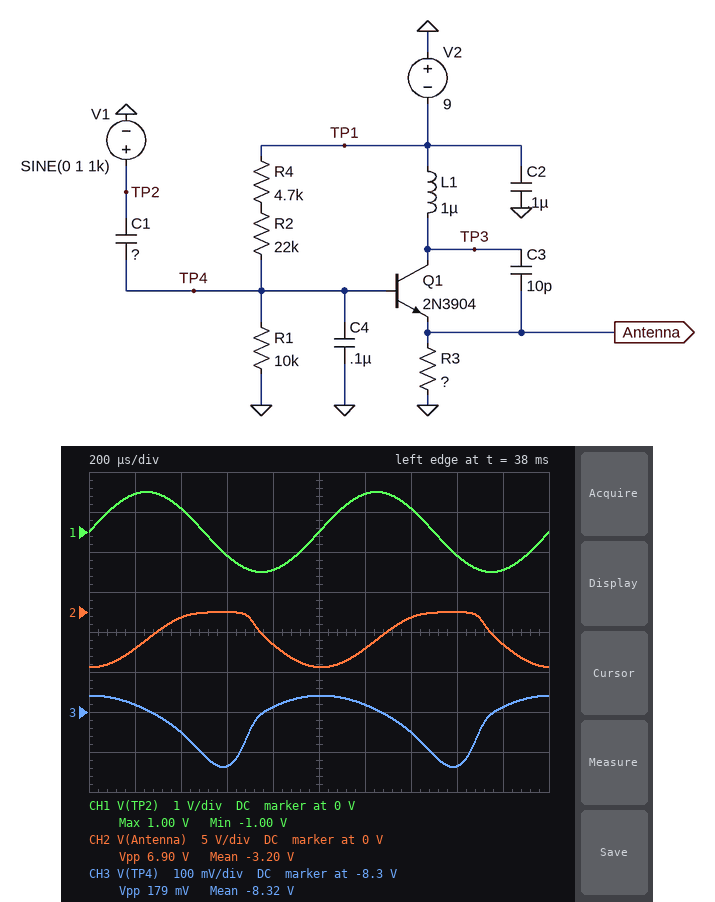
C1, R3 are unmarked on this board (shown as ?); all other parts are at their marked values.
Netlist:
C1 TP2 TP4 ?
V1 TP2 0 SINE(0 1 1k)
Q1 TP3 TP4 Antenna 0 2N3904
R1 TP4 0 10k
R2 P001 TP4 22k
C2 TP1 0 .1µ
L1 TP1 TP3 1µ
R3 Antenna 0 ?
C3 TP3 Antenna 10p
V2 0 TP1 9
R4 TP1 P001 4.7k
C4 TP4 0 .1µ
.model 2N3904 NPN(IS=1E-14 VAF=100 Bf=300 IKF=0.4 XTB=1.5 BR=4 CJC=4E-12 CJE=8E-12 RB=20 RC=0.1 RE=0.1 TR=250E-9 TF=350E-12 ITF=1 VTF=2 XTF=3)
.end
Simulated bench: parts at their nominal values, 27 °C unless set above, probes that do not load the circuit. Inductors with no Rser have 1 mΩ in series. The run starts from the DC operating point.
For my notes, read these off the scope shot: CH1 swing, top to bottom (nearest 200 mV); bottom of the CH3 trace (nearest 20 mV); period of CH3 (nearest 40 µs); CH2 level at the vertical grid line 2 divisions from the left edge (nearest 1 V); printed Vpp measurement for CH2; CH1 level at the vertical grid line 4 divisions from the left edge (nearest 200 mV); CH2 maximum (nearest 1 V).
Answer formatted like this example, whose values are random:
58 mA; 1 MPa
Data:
2.0 V; -8.44 V; 1.00 ms; -1 V; 6.90 V; -1.0 V; 0 V
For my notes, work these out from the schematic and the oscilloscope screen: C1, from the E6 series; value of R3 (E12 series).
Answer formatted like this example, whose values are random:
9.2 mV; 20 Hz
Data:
150 nF; 1 kΩ
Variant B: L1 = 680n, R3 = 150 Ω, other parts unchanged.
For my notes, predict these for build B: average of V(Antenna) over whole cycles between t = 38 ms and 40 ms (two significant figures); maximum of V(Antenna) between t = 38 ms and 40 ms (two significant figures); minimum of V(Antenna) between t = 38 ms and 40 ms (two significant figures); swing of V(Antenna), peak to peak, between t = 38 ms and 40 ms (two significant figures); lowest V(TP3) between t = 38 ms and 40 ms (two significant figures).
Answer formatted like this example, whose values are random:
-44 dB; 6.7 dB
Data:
-480 mV; -4.1 mV; -1.0 V; 1.0 V; -9.0 V
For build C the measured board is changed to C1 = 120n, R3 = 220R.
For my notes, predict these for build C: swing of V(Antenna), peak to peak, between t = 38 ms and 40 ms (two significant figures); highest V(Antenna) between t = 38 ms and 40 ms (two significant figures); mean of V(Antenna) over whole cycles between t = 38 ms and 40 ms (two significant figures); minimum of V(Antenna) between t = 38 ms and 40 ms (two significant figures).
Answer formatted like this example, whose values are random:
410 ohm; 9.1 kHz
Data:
1.3 V; -76 mV; -700 mV; -1.4 V
